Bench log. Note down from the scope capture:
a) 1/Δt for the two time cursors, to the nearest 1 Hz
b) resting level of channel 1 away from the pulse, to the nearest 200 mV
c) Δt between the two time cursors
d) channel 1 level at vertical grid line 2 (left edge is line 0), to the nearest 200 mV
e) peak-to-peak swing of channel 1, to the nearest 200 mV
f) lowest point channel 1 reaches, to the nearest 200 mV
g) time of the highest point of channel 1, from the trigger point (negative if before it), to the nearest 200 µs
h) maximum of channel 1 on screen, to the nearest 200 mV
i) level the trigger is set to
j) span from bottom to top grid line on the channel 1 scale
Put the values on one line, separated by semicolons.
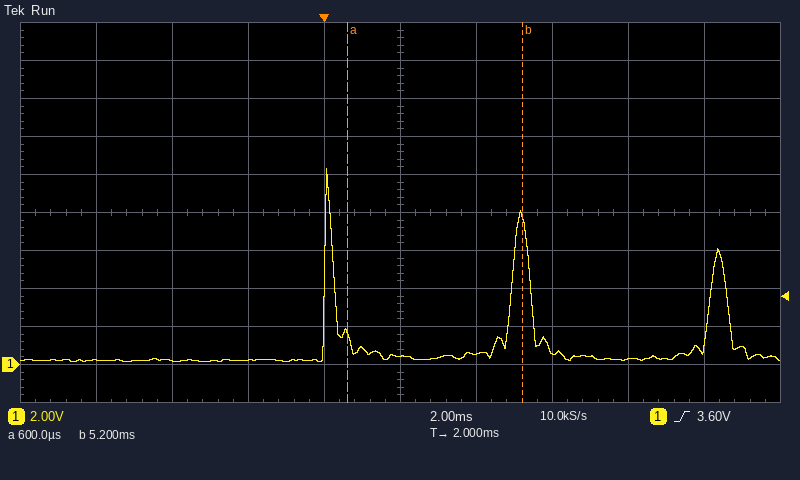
217 Hz; 200 mV; 4.6 ms; 200 mV; 10.2 V; 200 mV; 0.0 ms; 10.4 V; 3.60 V; 20 V
